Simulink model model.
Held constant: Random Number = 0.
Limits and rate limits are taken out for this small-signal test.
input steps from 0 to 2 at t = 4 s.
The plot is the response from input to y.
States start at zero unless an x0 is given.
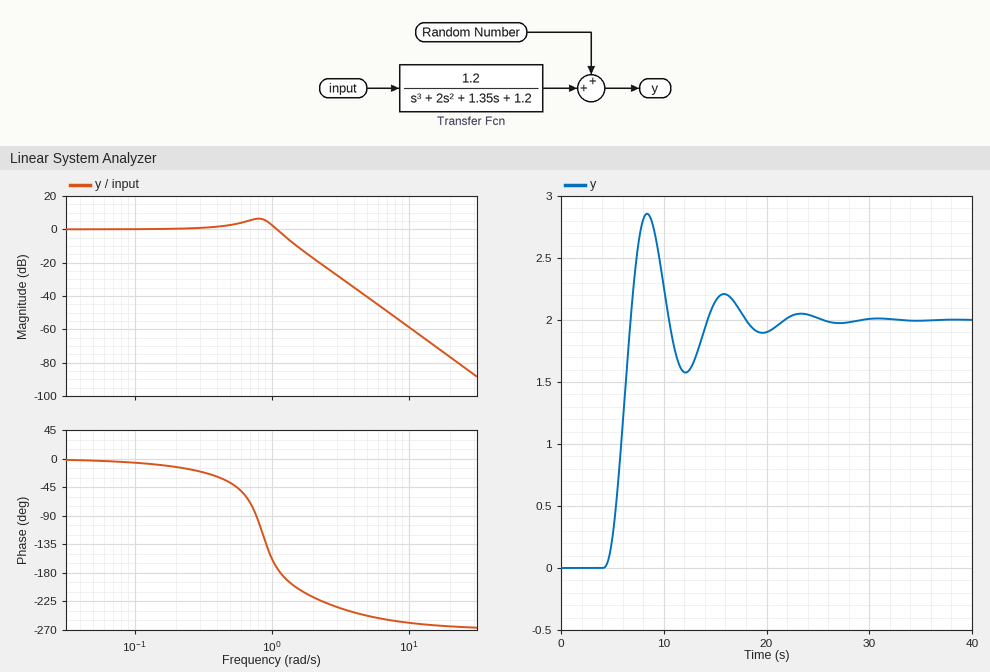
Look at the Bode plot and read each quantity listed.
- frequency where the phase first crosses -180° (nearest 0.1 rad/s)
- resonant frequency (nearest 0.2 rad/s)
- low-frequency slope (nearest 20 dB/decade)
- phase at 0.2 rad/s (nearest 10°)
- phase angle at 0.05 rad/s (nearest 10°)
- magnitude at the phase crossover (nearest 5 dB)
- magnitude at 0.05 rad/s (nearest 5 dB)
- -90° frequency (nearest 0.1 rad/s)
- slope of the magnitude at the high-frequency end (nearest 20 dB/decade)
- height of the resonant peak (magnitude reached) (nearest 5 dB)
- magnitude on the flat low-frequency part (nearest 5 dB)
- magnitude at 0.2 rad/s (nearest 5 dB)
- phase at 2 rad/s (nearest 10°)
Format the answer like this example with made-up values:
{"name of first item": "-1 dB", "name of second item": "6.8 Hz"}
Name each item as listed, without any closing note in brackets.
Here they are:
{"frequency where the phase first crosses -180°": "1.2 rad/s", "resonant frequency": "0.8 rad/s", "low-frequency slope": "0 dB/decade", "phase at 0.2 rad/s": "-10°", "phase angle at 0.05 rad/s": "0°", "magnitude at the phase crossover": "0 dB", "magnitude at 0.05 rad/s": "0 dB", "-90° frequency": "0.8 rad/s", "slope of the magnitude at the high-frequency end": "-60 dB/decade", "height of the resonant peak (magnitude reached)": "5 dB", "magnitude on the flat low-frequency part": "0 dB", "magnitude at 0.2 rad/s": "0 dB", "phase at 2 rad/s": "-220°"}
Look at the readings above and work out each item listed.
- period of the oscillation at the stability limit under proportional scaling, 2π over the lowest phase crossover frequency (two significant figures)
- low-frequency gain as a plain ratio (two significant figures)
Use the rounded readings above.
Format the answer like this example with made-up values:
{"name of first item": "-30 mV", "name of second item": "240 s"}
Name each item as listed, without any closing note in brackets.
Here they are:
{"period of the oscillation at the stability limit under proportional scaling, 2π over the lowest phase crossover frequency": "5.2 s", "low-frequency gain as a plain ratio": "1.0"}
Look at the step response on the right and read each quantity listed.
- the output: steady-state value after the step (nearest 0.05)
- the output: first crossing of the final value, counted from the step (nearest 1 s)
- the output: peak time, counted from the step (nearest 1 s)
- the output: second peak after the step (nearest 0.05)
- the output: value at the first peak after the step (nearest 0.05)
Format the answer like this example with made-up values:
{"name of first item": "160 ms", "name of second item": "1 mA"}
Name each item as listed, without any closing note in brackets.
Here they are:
{"the output: steady-state value after the step": "2.00", "the output: first crossing of the final value, counted from the step": "3 s", "the output: peak time, counted from the step": "4 s", "the output: second peak after the step": "2.20", "the output: value at the first peak after the step": "2.85"}
